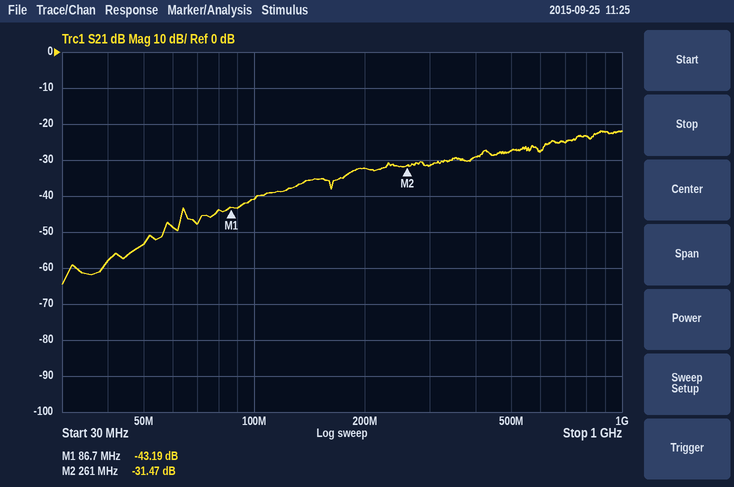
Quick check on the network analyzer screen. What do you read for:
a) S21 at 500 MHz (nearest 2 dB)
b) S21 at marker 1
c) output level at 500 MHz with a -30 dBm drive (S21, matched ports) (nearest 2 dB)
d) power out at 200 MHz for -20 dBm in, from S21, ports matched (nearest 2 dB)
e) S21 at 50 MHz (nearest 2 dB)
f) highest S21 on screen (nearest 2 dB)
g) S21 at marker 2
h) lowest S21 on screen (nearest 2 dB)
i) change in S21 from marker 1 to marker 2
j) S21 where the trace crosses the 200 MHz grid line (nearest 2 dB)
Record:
-28 dB
-43.19 dB
-58 dBm
-52 dBm
-54 dB
-22 dB
-31.47 dB
-64 dB
11.72 dB
-32 dB
